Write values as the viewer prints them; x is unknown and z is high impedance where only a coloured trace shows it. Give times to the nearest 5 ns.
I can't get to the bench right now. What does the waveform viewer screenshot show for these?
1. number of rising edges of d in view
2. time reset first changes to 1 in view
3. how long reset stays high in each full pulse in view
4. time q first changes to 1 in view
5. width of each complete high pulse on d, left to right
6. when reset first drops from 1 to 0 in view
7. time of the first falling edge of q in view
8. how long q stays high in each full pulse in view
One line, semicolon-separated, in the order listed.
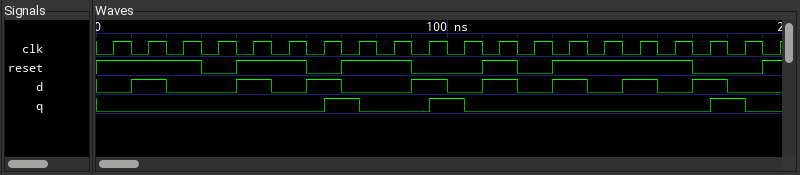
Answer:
8; 40 ns; 20 ns, 20 ns, 10 ns, 40 ns; 65 ns; 10 ns, 10 ns, 10 ns, 10 ns, 10 ns, 10 ns, 10 ns, 10 ns; 30 ns; 75 ns; 10 ns, 10 ns, 10 ns
